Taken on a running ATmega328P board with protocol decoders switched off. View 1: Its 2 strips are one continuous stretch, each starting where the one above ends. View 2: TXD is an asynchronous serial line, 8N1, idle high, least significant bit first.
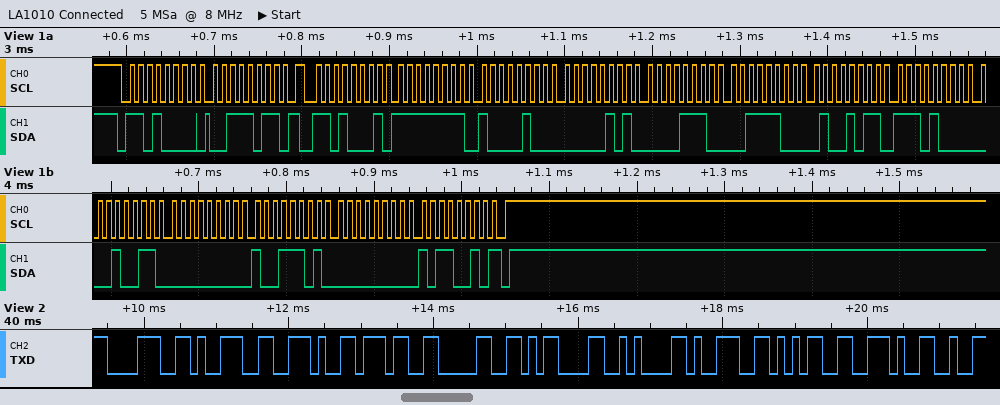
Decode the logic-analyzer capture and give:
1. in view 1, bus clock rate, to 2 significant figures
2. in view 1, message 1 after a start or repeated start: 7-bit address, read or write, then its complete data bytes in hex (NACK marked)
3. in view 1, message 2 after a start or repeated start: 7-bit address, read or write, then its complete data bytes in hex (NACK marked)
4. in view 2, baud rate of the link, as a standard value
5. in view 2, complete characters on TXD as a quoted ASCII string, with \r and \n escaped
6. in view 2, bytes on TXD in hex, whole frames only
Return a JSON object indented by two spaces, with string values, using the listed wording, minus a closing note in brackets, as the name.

{
  "in view 1, bus clock rate, to 2 significant figures": "100 kHz",
  "in view 1, message 1 after a start or repeated start: 7-bit address, read or write, then its complete data bytes in hex": "0x68 write: 3B",
  "in view 1, message 2 after a start or repeated start: 7-bit address, read or write, then its complete data bytes in hex": "0x68 read: FF 84 05 0E 3C 4B E8 13 00 9D 00 B2 NACK",
  "in view 2, baud rate of the link, as a standard value": "9600 baud",
  "in view 2, complete characters on TXD as a quoted ASCII string, with \\r and \\n escaped": "\"89.70\\r\\n95.\"",
  "in view 2, bytes on TXD in hex, whole frames only": "38 39 2E 37 30 0D 0A 39 35 2E"
}
